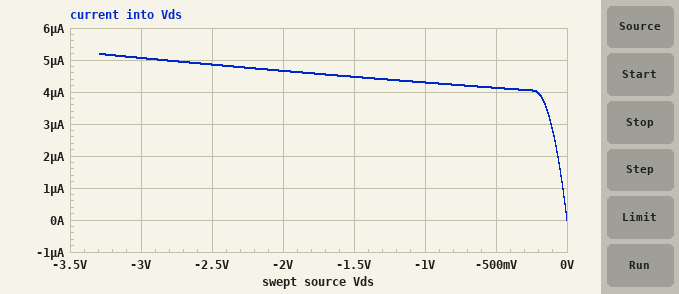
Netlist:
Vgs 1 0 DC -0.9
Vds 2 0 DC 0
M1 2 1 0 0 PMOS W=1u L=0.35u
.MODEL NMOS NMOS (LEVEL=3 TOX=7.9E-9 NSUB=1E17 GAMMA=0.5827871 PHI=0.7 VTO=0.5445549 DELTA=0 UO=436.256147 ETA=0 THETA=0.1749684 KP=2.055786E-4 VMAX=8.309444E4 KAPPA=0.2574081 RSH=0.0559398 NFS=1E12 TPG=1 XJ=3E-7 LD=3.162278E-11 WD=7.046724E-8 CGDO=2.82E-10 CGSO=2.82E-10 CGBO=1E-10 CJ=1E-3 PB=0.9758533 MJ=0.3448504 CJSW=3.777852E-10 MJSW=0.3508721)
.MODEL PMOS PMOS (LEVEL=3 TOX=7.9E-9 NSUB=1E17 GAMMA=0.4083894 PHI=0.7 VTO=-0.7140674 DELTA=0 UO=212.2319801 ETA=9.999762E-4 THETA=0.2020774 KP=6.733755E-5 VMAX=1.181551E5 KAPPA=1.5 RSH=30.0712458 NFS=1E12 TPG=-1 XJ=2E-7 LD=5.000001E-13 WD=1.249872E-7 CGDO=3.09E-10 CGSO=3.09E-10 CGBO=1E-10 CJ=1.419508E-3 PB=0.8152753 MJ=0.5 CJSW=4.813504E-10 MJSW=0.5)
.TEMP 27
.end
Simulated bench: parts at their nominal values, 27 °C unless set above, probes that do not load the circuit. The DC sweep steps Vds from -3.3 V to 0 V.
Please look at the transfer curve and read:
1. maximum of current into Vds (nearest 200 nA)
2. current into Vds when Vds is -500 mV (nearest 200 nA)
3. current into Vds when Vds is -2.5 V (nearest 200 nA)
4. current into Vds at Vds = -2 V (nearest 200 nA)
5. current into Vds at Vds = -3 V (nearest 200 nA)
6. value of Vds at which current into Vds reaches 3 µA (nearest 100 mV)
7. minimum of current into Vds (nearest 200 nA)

5.2 µA
4.2 µA
4.8 µA
4.6 µA
5.0 µA
-100 mV
0 A
